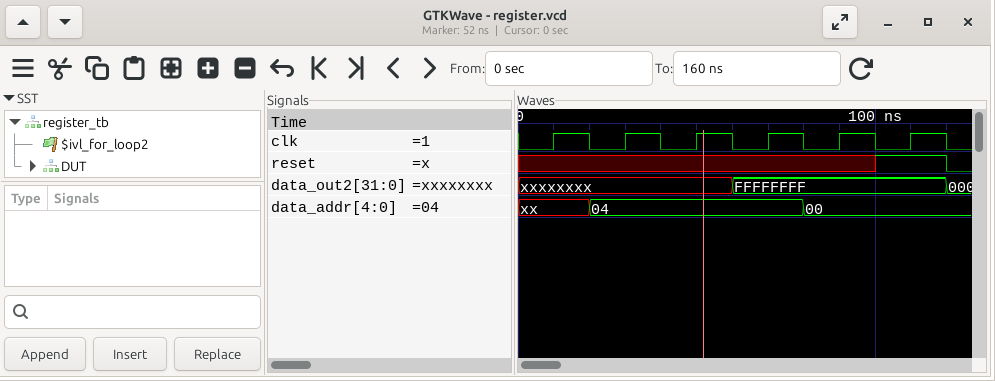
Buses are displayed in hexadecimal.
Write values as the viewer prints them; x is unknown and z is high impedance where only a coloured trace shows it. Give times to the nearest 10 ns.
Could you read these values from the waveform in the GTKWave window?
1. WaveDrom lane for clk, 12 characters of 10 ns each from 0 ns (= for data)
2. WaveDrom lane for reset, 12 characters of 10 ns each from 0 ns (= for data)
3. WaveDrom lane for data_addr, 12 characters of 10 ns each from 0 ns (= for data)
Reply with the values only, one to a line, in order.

{name: 'clk', wave: '010101010101'}
{name: 'reset', wave: 'x.........1.'}
{name: 'data_addr', wave: 'x.=.....=...', data: '04 00'}
